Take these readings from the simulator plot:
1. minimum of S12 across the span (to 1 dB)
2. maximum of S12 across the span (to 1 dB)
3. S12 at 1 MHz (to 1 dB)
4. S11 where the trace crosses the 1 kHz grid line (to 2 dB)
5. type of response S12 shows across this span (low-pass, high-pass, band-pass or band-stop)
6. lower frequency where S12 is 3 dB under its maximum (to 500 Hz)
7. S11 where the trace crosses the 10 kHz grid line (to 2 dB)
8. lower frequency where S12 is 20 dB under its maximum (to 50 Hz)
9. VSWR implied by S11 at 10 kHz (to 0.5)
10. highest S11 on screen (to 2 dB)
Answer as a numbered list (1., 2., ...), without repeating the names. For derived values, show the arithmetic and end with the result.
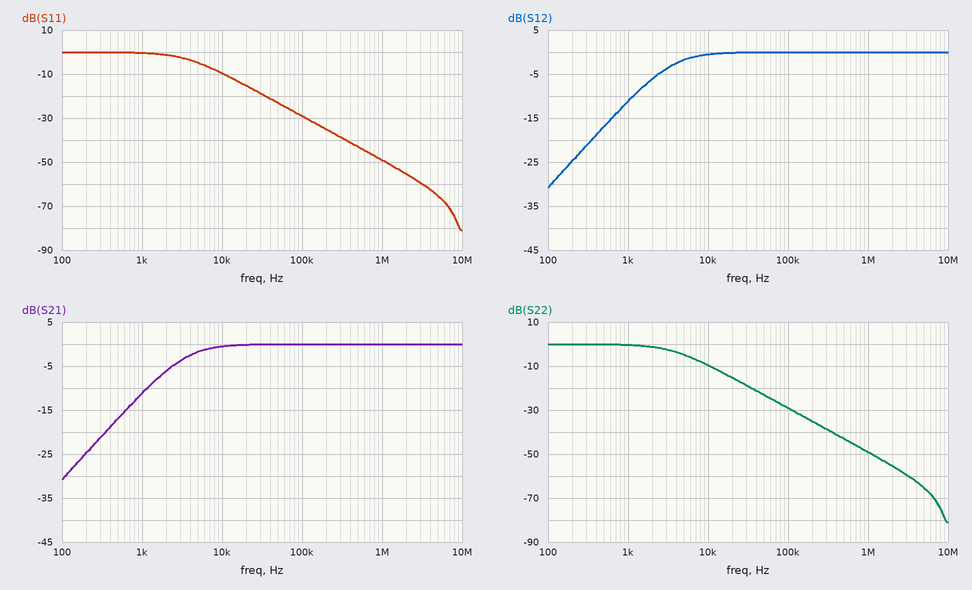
1. -31 dB
2. 0 dB
3. 0 dB
4. 0 dB
5. high-pass
6. 3.5 kHz
7. -10 dB
8. 350 Hz
9. |Γ| = 10^(-10/20) = 0.3162; VSWR = (1 + 0.3162)/(1 − 0.3162) ≈ 1.92, so 2.0 to the nearest 0.5
10. 0 dB
